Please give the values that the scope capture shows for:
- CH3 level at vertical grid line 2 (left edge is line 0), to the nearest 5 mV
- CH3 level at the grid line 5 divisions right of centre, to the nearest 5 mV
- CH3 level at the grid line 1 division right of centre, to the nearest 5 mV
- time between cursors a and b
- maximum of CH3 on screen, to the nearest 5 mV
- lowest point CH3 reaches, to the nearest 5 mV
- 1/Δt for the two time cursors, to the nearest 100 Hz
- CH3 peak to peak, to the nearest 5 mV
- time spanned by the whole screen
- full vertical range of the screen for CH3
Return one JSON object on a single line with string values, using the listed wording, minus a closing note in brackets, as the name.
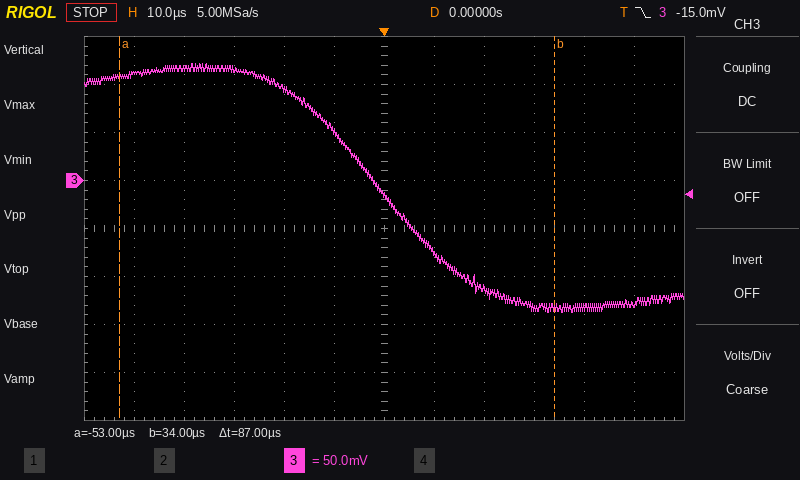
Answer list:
{"CH3 level at vertical grid line 2 (left edge is line 0), to the nearest 5 mV": "115 mV", "CH3 level at the grid line 5 divisions right of centre, to the nearest 5 mV": "-130 mV", "CH3 level at the grid line 1 division right of centre, to the nearest 5 mV": "-75 mV", "time between cursors a and b": "87 µs", "maximum of CH3 on screen, to the nearest 5 mV": "120 mV", "lowest point CH3 reaches, to the nearest 5 mV": "-140 mV", "1/Δt for the two time cursors, to the nearest 100 Hz": "11.5 kHz", "CH3 peak to peak, to the nearest 5 mV": "260 mV", "time spanned by the whole screen": "120 µs", "full vertical range of the screen for CH3": "400 mV"}
